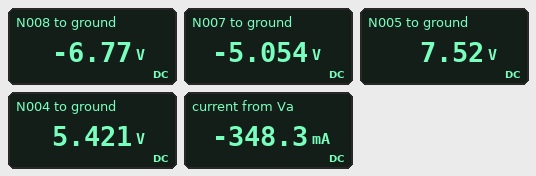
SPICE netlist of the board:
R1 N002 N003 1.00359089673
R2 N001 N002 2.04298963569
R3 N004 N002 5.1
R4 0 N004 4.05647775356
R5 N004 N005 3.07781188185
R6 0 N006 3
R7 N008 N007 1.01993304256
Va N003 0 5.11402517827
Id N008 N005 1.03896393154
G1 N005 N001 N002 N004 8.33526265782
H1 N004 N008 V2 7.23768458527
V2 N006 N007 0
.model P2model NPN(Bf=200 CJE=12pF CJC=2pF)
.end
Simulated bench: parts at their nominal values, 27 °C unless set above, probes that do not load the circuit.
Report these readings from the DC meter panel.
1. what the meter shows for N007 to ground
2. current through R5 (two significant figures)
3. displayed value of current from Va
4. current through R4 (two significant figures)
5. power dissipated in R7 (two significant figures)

-5.054 V
680 mA
-348.3 mA
1.3 A
2.9 W
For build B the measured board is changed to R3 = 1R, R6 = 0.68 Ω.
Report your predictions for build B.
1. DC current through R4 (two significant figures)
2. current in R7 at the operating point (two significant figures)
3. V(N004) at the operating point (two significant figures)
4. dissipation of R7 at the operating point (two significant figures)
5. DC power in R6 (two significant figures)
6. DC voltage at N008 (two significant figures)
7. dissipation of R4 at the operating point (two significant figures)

1.2 A
870 mA
4.8 V
780 mW
520 mW
-1.5 V
5.8 W
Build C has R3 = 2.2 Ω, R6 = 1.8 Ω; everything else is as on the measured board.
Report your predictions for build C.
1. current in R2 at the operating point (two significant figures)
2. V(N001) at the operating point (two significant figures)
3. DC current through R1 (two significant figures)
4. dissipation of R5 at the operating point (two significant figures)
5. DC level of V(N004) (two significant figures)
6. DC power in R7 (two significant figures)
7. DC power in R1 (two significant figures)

110 mA
4.8 V
100 mA
4.0 W
5.0 V
1.3 W
10 mW
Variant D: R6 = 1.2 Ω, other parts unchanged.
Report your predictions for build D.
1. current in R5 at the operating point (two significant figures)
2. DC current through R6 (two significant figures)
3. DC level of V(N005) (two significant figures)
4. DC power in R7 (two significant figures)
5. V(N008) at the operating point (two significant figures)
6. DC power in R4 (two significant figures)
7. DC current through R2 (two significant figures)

1.3 A
980 mA
8.8 V
980 mW
-2.2 V
5.9 W
240 mA
